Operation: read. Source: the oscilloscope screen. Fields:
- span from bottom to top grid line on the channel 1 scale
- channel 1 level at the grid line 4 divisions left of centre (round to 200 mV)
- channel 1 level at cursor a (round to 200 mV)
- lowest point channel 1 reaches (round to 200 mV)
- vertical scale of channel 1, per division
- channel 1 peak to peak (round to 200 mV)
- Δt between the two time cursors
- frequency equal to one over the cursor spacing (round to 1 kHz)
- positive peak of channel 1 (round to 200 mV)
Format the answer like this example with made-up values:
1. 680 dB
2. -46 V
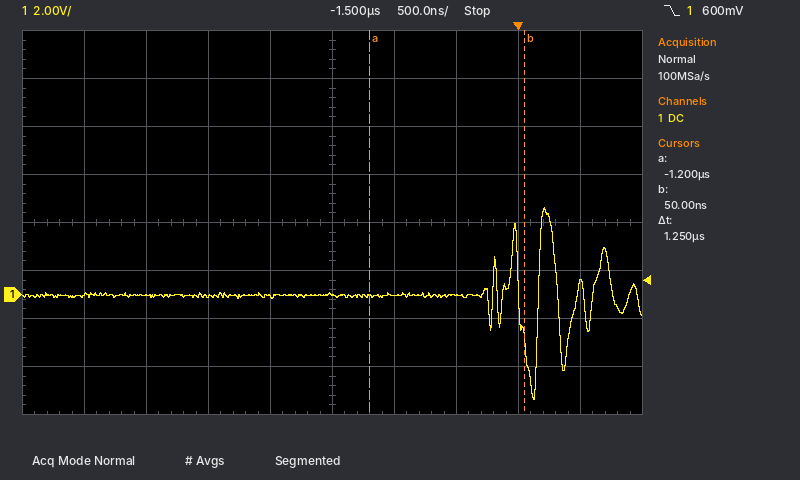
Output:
1. 16 V
2. 0.0 V
3. 0.0 V
4. -4.4 V
5. 2 V
6. 8.0 V
7. 1.25 µs
8. 800 kHz
9. 3.6 V
